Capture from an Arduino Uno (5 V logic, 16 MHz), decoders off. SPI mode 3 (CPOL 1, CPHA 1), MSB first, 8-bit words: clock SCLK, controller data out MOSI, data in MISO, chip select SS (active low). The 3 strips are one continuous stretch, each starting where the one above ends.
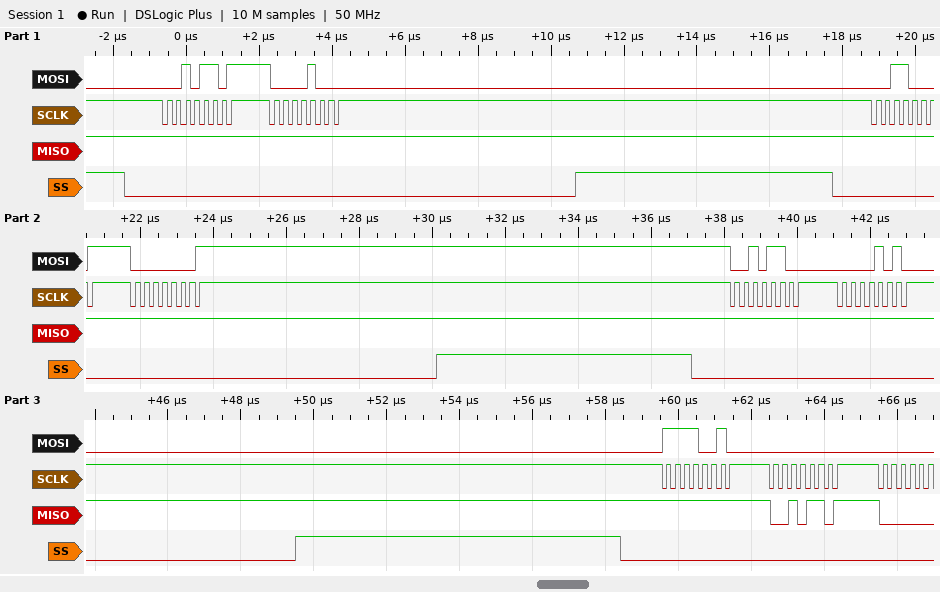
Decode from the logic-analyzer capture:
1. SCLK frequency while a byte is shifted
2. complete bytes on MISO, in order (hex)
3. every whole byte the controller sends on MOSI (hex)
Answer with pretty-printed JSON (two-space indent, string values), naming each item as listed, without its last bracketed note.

{
  "SCLK frequency while a byte is shifted": "4 MHz",
  "complete bytes on MISO, in order": "FF FF FF FF FF FF FF 2D",
  "every whole byte the controller sends on MOSI": "2D 08 31 01 2C 0A F2 00"
}
